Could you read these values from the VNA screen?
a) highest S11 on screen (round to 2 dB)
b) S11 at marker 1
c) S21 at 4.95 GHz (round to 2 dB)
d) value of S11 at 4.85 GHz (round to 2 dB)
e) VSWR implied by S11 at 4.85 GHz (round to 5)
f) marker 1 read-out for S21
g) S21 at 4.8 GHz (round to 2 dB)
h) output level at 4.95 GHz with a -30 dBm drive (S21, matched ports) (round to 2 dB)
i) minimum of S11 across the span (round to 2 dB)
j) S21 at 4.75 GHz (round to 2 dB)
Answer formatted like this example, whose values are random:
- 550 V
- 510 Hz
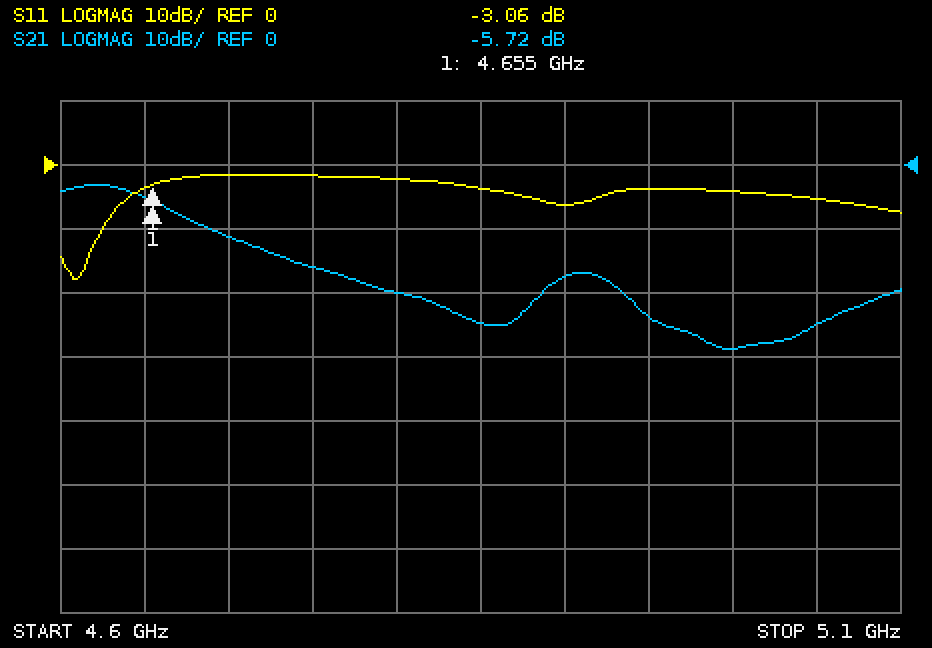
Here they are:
- -2 dB
- -3.06 dB
- -24 dB
- -4 dB
- 5
- -5.72 dB
- -20 dB
- -54 dBm
- -18 dB
- -16 dB
